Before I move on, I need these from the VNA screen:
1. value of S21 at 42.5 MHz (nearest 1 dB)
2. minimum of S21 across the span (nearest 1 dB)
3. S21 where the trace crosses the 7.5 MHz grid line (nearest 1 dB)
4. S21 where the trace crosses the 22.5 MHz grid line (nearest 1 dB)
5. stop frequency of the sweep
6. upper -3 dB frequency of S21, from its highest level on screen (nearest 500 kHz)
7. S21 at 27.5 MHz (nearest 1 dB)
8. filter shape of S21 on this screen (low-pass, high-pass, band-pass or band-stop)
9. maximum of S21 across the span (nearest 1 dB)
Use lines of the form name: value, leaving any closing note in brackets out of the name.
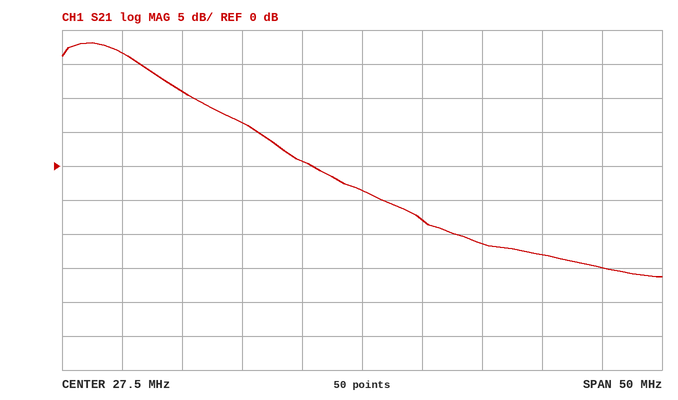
value of S21 at 42.5 MHz: -13 dB
minimum of S21 across the span: -16 dB
S21 where the trace crosses the 7.5 MHz grid line: 17 dB
S21 where the trace crosses the 22.5 MHz grid line: 1 dB
stop frequency of the sweep: 52.5 MHz
upper -3 dB frequency of S21, from its highest level on screen: 9.0 MHz
S21 at 27.5 MHz: -4 dB
filter shape of S21 on this screen: low-pass
maximum of S21 across the span: 18 dB
